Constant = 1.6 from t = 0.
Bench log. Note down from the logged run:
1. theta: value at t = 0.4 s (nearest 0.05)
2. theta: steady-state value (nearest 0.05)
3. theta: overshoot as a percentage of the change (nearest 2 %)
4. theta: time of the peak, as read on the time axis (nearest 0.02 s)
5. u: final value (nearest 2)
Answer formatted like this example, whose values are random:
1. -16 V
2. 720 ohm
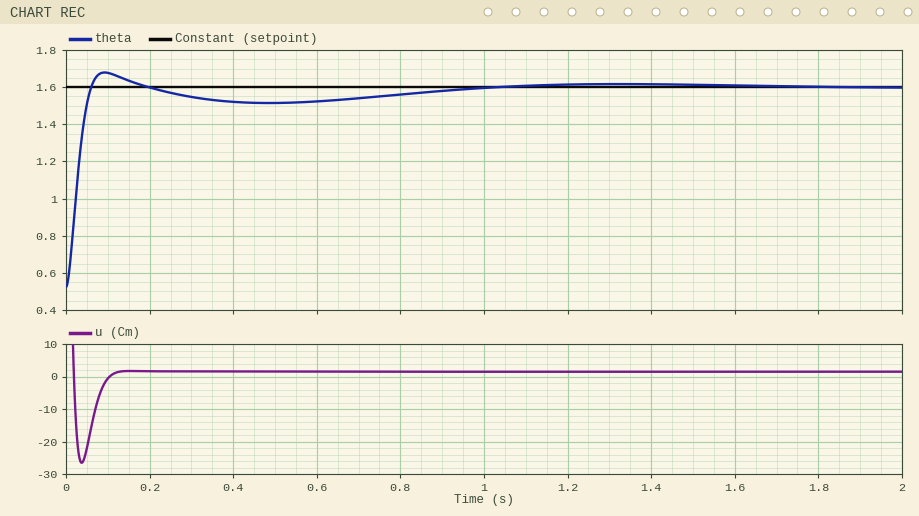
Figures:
1. 1.50
2. 1.60
3. 8 %
4. 0.10 s
5. 2
